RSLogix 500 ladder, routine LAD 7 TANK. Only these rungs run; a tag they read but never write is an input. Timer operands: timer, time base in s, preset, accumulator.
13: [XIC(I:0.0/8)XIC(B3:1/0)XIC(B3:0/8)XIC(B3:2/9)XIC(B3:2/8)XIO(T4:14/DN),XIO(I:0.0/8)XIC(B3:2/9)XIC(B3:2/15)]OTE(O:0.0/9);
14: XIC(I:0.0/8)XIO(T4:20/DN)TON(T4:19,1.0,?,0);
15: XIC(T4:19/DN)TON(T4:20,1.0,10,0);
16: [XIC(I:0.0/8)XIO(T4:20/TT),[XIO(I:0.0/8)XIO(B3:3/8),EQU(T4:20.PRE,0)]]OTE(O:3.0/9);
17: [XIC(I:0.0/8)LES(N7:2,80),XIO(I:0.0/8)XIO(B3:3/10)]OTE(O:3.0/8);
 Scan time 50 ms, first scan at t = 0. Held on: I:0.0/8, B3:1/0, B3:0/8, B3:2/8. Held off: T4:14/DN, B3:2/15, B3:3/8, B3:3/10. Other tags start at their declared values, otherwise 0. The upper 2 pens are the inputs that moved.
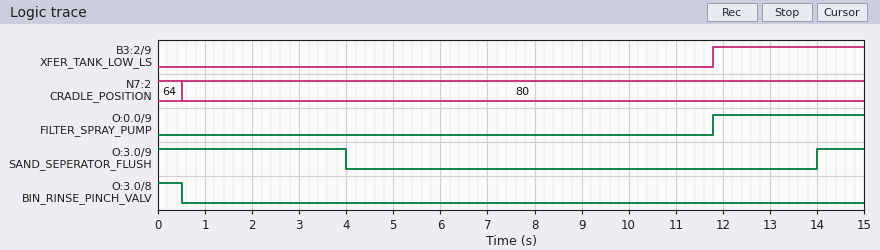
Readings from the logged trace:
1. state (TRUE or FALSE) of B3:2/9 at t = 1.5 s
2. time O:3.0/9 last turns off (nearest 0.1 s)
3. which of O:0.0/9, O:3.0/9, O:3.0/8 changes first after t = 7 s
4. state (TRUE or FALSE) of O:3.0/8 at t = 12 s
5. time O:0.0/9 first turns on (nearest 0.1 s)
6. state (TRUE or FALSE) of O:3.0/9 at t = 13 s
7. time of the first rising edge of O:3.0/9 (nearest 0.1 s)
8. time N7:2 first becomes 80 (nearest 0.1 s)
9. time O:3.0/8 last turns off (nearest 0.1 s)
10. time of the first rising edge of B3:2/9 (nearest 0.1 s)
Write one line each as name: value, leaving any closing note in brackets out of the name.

state (TRUE or FALSE) of B3:2/9 at t = 1.5 s: FALSE
time O:3.0/9 last turns off: 4.0 s
which of O:0.0/9, O:3.0/9, O:3.0/8 changes first after t = 7 s: O:0.0/9
state (TRUE or FALSE) of O:3.0/8 at t = 12 s: FALSE
time O:0.0/9 first turns on: 11.8 s
state (TRUE or FALSE) of O:3.0/9 at t = 13 s: FALSE
time of the first rising edge of O:3.0/9: 14.0 s
time N7:2 first becomes 80: 0.5 s
time O:3.0/8 last turns off: 0.5 s
time of the first rising edge of B3:2/9: 11.8 s
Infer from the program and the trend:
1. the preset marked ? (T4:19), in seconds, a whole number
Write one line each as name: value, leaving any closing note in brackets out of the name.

the preset marked ? (T4:19), in seconds, a whole number: 4 s
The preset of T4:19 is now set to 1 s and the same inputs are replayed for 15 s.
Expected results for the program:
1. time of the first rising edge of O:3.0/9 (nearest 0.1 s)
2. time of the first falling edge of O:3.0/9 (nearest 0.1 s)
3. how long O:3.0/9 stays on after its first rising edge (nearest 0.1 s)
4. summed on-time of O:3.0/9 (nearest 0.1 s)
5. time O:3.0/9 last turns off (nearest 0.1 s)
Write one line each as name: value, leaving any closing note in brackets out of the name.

time of the first rising edge of O:3.0/9: 11.0 s
time of the first falling edge of O:3.0/9: 1.0 s
how long O:3.0/9 stays on after its first rising edge: 1.1 s
summed on-time of O:3.0/9: 2.1 s
time O:3.0/9 last turns off: 12.1 s
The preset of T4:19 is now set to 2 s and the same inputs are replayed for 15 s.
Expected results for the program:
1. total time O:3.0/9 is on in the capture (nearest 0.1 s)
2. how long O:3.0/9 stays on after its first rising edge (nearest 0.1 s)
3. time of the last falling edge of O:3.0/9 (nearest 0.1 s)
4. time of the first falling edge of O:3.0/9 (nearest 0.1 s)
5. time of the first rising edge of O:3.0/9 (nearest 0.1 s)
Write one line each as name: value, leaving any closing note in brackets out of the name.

total time O:3.0/9 is on in the capture: 4.1 s
how long O:3.0/9 stays on after its first rising edge: 2.1 s
time of the last falling edge of O:3.0/9: 14.1 s
time of the first falling edge of O:3.0/9: 2.0 s
time of the first rising edge of O:3.0/9: 12.0 s
